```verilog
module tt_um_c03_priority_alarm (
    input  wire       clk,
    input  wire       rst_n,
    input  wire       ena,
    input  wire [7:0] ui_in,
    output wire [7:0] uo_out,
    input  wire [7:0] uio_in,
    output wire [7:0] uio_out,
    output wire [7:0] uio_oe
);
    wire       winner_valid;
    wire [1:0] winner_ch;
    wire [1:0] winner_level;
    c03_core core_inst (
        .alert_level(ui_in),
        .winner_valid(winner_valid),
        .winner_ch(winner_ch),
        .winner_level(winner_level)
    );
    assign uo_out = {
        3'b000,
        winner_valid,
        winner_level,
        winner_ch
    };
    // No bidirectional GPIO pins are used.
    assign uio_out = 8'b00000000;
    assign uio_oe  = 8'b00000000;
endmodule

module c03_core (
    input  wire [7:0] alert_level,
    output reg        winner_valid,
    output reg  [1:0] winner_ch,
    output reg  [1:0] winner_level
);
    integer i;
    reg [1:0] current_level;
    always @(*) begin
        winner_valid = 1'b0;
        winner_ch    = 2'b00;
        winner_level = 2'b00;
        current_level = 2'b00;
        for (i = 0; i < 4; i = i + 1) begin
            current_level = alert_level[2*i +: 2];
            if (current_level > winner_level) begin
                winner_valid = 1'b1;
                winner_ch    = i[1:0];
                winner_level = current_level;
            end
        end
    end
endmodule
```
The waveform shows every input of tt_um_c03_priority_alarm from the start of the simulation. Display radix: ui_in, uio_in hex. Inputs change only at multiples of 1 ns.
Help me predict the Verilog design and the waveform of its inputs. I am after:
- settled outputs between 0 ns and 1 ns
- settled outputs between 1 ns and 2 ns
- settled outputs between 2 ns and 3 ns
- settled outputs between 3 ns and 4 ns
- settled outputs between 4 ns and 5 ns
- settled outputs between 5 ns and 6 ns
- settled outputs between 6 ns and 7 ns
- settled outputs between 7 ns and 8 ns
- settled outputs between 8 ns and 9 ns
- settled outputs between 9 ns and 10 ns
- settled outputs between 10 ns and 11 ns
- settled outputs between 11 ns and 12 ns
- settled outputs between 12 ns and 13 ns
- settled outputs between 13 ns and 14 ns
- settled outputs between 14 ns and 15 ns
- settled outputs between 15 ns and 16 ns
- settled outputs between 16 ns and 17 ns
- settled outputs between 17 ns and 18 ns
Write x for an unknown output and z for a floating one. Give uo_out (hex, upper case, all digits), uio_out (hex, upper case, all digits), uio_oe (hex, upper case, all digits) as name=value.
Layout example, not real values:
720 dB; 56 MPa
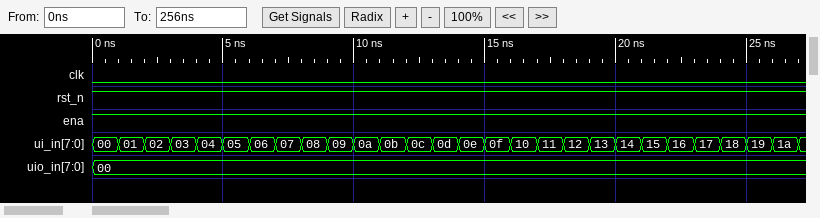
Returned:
uo_out=00, uio_out=00, uio_oe=00; uo_out=14, uio_out=00, uio_oe=00; uo_out=18, uio_out=00, uio_oe=00; uo_out=1C, uio_out=00, uio_oe=00; uo_out=15, uio_out=00, uio_oe=00; uo_out=14, uio_out=00, uio_oe=00; uo_out=18, uio_out=00, uio_oe=00; uo_out=1C, uio_out=00, uio_oe=00; uo_out=19, uio_out=00, uio_oe=00; uo_out=19, uio_out=00, uio_oe=00; uo_out=18, uio_out=00, uio_oe=00; uo_out=1C, uio_out=00, uio_oe=00; uo_out=1D, uio_out=00, uio_oe=00; uo_out=1D, uio_out=00, uio_oe=00; uo_out=1D, uio_out=00, uio_oe=00; uo_out=1C, uio_out=00, uio_oe=00; uo_out=16, uio_out=00, uio_oe=00; uo_out=14, uio_out=00, uio_oe=00
